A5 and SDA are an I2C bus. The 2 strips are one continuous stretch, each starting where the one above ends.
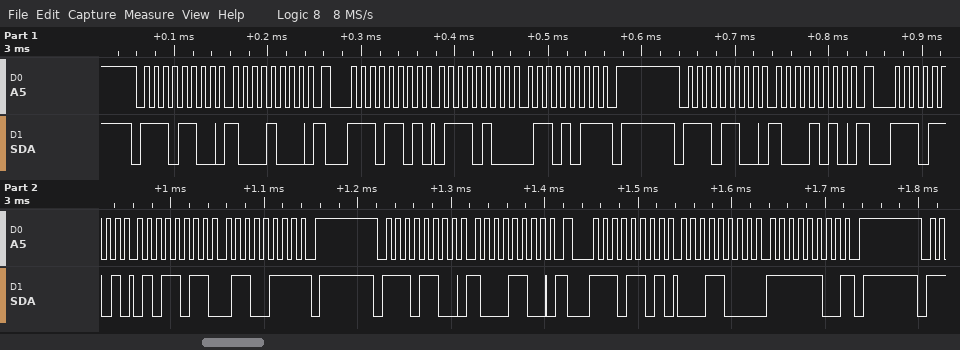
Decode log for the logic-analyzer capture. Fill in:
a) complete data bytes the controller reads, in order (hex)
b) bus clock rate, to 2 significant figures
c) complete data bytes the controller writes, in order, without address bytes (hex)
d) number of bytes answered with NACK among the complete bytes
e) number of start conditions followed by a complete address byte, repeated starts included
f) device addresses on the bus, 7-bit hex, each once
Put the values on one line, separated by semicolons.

74 6B 5B 67 18 FC; 100 kHz; 88 8A 8C; 3; 6; 0x76
